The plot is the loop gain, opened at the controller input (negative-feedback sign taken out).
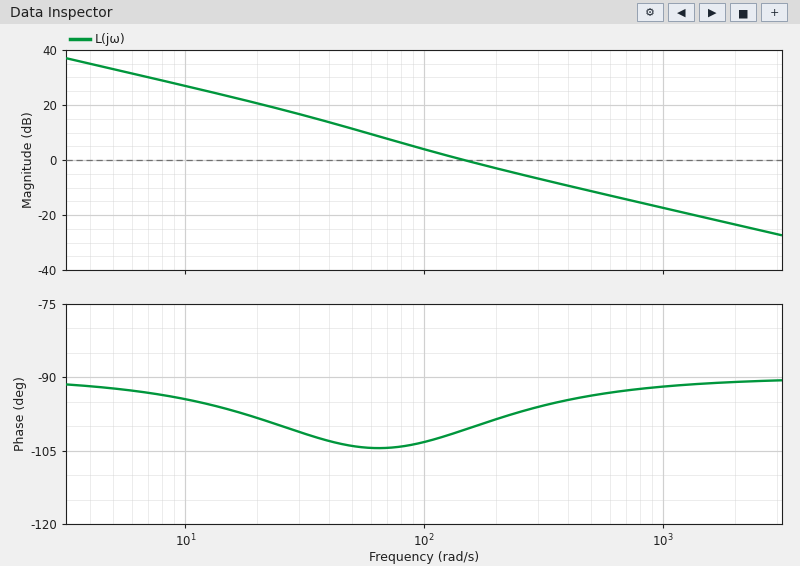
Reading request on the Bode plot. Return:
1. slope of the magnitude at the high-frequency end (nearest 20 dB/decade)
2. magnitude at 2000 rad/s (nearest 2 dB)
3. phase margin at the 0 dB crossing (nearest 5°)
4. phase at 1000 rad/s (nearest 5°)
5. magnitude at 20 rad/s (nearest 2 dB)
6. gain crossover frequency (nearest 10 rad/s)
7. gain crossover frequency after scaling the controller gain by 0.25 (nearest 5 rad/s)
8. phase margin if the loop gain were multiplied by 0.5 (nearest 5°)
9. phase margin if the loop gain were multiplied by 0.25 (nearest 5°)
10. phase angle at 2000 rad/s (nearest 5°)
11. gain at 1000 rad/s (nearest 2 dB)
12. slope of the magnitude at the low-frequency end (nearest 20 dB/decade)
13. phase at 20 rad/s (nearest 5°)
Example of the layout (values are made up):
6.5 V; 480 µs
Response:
-20 dB/decade; -24 dB; 80°; -90°; 20 dB; 150 rad/s; 45 rad/s; 75°; 75°; -90°; -18 dB; -20 dB/decade; -100°
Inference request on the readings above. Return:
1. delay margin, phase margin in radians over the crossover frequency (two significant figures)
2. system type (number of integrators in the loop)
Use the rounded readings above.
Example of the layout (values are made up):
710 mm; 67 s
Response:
0.0093 s; 1
